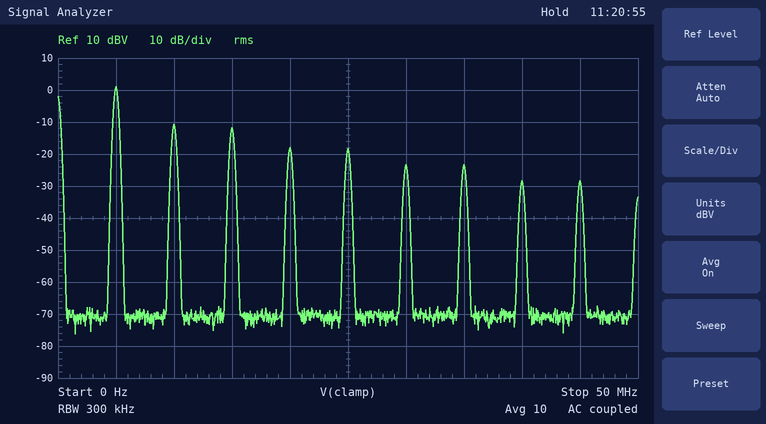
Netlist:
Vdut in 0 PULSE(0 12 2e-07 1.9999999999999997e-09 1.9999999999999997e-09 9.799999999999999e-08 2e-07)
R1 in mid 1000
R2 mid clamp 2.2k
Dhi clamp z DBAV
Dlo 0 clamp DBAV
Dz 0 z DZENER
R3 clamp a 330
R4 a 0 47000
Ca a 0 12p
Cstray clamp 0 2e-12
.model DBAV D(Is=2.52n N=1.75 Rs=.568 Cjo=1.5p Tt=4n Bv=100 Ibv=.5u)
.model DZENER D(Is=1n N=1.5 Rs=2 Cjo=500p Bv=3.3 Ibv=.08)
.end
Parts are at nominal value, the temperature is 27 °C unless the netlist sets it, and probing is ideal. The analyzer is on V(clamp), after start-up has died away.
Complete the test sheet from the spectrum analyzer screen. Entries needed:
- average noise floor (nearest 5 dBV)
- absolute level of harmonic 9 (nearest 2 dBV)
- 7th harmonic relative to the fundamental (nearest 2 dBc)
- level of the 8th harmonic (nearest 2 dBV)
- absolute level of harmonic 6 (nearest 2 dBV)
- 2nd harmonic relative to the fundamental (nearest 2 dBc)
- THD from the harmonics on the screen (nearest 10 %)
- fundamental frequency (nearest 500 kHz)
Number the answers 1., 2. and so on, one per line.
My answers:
1. -70 dBV
2. -28 dBV
3. -24 dBc
4. -28 dBV
5. -24 dBV
6. -12 dBc
7. 40 %
8. 5.0 MHz
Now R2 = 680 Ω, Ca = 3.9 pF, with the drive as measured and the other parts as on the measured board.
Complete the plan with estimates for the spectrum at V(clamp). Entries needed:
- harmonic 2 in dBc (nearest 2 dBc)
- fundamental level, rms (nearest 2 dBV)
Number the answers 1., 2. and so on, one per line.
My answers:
1. -14 dBc
2. 4 dBV
